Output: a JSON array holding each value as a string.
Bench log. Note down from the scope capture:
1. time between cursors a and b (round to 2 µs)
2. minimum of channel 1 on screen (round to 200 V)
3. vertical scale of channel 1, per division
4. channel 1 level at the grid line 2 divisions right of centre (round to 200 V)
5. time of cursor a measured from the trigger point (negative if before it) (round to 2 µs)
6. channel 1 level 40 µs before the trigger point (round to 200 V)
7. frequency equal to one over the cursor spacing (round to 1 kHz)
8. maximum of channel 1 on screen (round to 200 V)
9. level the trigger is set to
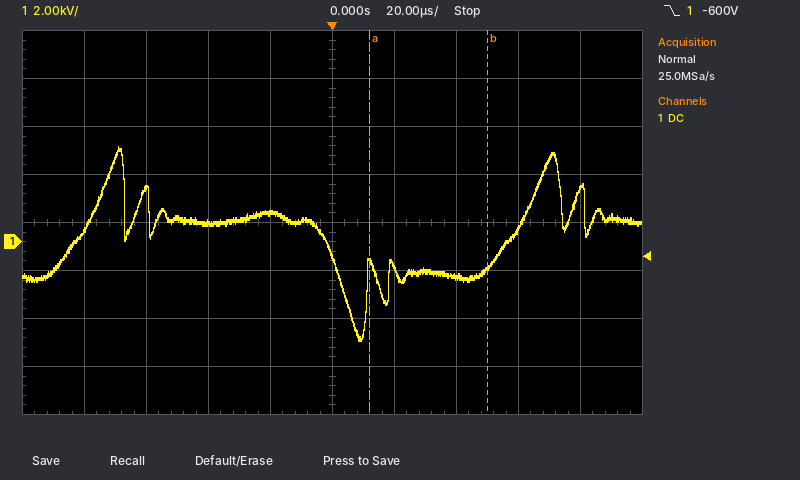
["38 µs", "-4.2 kV", "2 kV", "-1.4 kV", "+12 µs", "800 V", "26 kHz", "4.0 kV", "-600 V"]
